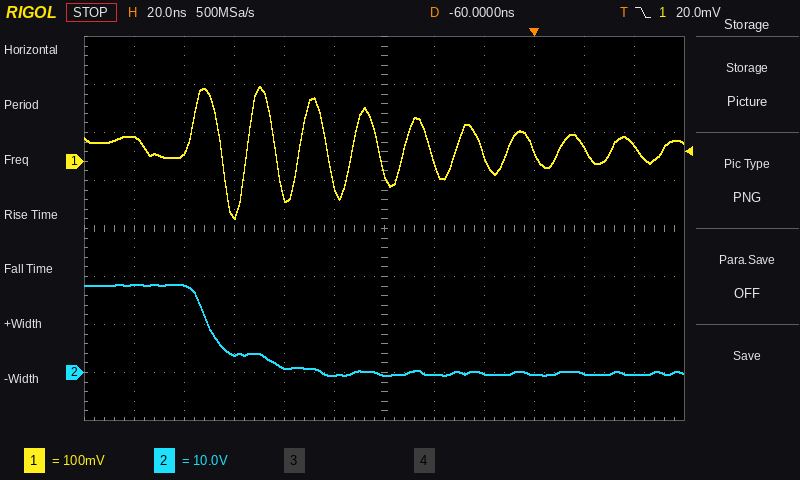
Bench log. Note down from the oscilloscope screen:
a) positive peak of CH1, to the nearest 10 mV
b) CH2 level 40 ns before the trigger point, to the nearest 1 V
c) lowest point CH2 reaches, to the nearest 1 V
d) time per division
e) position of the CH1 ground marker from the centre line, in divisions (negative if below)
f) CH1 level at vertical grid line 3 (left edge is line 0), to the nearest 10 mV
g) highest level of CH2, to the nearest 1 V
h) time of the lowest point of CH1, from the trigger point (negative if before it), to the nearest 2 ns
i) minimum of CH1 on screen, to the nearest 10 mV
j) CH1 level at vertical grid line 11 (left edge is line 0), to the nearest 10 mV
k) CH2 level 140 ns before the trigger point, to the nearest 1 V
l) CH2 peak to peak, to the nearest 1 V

160 mV
0 V
-1 V
20 ns
+1.4 div
-110 mV
18 V
-120 ns
-120 mV
30 mV
18 V
19 V
